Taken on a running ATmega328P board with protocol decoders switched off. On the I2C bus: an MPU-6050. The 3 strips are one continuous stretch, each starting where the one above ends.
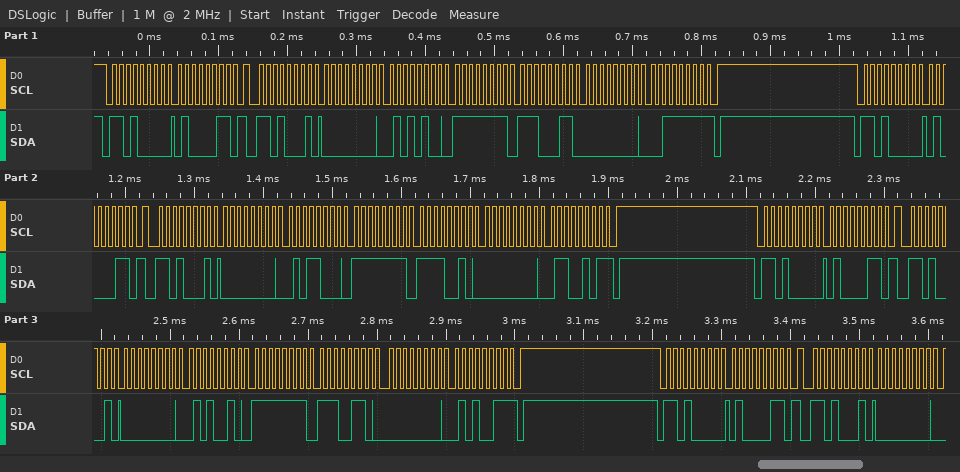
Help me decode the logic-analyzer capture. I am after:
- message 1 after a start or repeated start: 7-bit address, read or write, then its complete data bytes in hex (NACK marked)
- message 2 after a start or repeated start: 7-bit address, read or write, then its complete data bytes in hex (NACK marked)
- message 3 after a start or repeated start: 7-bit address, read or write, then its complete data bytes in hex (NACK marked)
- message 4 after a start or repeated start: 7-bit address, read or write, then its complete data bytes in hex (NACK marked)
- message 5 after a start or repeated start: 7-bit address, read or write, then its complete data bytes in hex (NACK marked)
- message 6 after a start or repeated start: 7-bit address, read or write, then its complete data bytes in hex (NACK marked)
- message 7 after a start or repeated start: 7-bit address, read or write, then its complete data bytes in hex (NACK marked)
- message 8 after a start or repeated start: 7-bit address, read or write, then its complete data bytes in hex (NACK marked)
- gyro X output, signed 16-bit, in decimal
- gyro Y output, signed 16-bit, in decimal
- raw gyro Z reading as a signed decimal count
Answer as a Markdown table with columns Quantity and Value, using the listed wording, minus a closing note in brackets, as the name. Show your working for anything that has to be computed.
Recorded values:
| Quantity | Value |
|---|---|
| message 1 after a start or repeated start: 7-bit address, read or write, then its complete data bytes in hex | 0x68 write: 43 |
| message 2 after a start or repeated start: 7-bit address, read or write, then its complete data bytes in hex | 0x68 read: 00 54 FF E3 00 3F NACK |
| message 3 after a start or repeated start: 7-bit address, read or write, then its complete data bytes in hex | 0x68 write: 43 |
| message 4 after a start or repeated start: 7-bit address, read or write, then its complete data bytes in hex | 0x68 read: 00 58 FF F2 00 65 NACK |
| message 5 after a start or repeated start: 7-bit address, read or write, then its complete data bytes in hex | 0x68 write: 43 |
| message 6 after a start or repeated start: 7-bit address, read or write, then its complete data bytes in hex | 0x68 read: 00 52 FF E6 00 53 NACK |
| message 7 after a start or repeated start: 7-bit address, read or write, then its complete data bytes in hex | 0x68 write: 43 |
| message 8 after a start or repeated start: 7-bit address, read or write, then its complete data bytes in hex | 0x68 read: 00 |
| gyro X output, signed 16-bit, in decimal | 0x0054 = 84 |
| gyro Y output, signed 16-bit, in decimal | 0xFFE3 = -29 |
| raw gyro Z reading as a signed decimal count | 0x003F = 63 |
